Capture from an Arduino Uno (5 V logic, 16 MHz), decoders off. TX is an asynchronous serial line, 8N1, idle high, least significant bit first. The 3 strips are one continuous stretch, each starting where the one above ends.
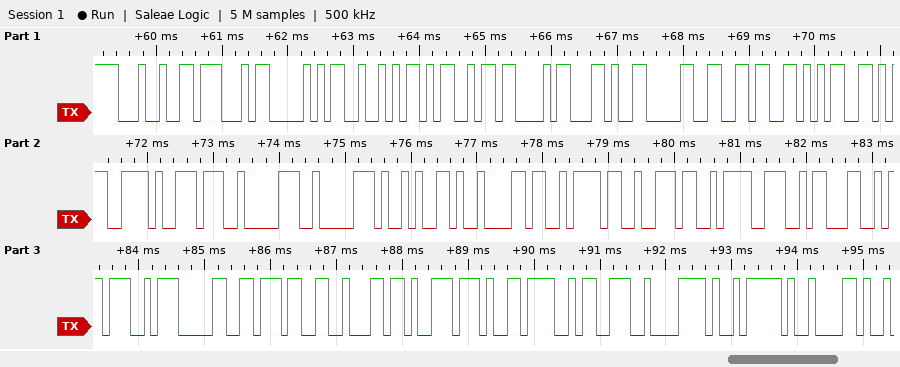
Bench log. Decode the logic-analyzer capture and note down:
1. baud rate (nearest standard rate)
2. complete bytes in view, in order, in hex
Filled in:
9600 baud
24 47 50 52 4D 43 2C 30 36 35 CD B9 82 82 29 09 D3 93 D3 4E 4C A7 30 37 62 B9 D9 9A C2 E9 09
